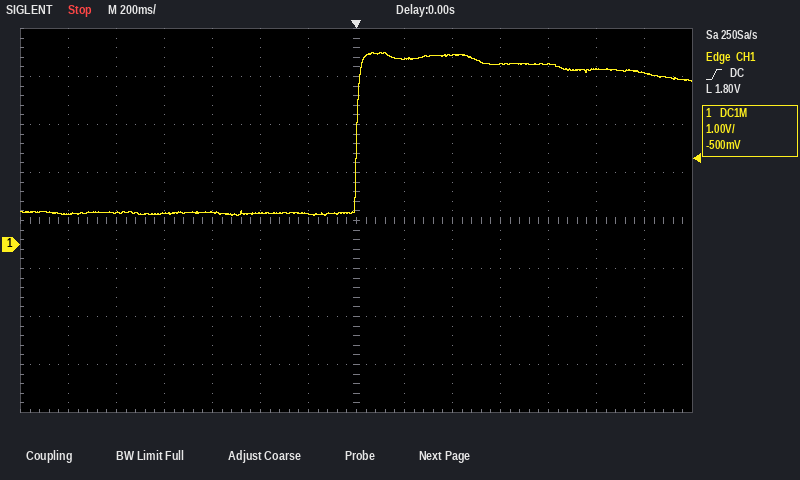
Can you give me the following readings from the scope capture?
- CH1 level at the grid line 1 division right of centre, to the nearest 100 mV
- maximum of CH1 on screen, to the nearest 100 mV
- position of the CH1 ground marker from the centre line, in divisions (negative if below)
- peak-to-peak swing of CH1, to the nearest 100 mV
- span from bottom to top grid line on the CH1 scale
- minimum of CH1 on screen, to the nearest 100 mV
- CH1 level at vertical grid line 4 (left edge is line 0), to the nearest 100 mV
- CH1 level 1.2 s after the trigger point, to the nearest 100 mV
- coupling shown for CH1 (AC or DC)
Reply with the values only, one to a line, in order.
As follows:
3.9 V
4.0 V
-0.5 div
3.4 V
8 V
600 mV
700 mV
3.6 V
DC
